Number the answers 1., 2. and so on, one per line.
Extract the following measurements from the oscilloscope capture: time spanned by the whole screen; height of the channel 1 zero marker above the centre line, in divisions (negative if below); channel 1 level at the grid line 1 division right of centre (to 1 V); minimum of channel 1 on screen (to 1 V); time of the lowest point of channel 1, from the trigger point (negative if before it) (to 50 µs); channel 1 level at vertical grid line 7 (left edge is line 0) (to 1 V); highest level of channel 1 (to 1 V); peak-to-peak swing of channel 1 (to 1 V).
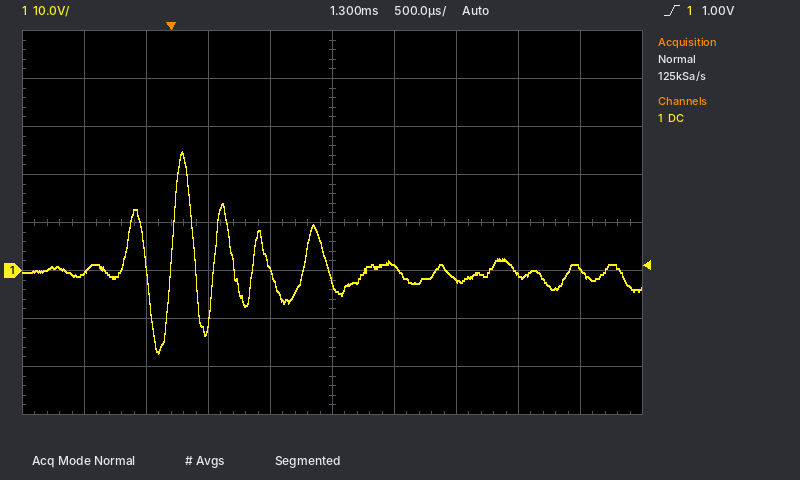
1. 5 ms
2. -1.0 div
3. 1 V
4. -17 V
5. -100 µs
6. -2 V
7. 25 V
8. 42 V
